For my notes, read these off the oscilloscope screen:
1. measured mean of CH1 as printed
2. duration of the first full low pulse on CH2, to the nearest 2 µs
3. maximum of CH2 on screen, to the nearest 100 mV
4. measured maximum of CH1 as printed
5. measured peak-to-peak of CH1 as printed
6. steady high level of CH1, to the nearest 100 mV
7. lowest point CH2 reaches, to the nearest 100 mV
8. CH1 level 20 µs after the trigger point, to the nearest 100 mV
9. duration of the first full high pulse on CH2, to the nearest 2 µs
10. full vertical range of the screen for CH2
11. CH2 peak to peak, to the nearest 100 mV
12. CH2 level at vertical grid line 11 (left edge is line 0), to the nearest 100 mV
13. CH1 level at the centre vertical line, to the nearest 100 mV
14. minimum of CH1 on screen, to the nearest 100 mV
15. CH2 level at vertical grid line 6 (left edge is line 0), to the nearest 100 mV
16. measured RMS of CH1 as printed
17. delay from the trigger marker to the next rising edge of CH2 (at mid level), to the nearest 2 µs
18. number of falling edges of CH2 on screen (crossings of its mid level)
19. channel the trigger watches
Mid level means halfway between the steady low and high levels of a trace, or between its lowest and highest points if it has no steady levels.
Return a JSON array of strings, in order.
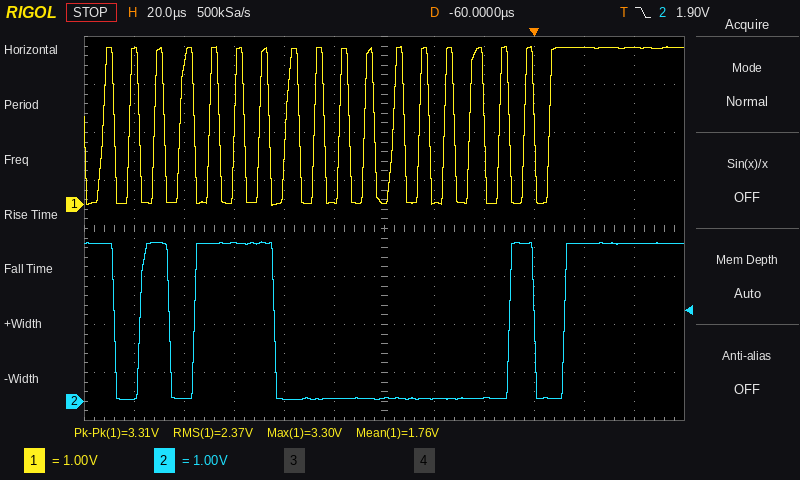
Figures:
["1.76 V", "10 µs", "3.3 V", "3.30 V", "3.31 V", "3.3 V", "0.0 V", "3.3 V", "12 µs", "8 V", "3.3 V", "3.3 V", "0.0 V", "0.0 V", "100 mV", "2.37 V", "12 µs", "4", "CH2"]
